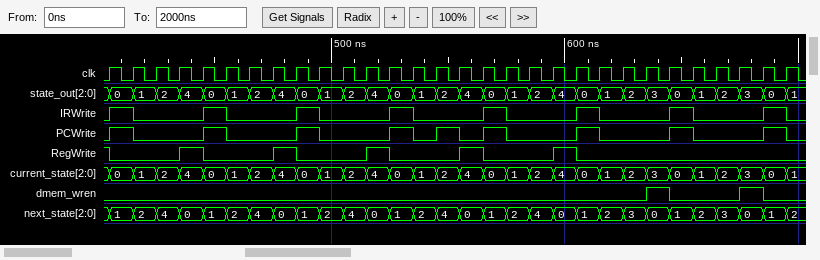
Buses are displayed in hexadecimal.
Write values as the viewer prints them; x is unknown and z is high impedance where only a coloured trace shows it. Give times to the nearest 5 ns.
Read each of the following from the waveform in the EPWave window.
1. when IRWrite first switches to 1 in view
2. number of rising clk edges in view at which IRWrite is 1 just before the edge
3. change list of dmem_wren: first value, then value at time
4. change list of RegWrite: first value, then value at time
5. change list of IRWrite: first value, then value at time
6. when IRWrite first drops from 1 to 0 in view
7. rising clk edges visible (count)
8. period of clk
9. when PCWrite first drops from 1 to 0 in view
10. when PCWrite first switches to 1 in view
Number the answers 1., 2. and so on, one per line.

1. 405 ns
2. 8
3. 0, 1 at 635 ns, 0 at 645 ns, 1 at 675 ns, 0 at 685 ns
4. 1, 0 at 405 ns, 1 at 435 ns, 0 at 445 ns, 1 at 475 ns, 0 at 485 ns, 1 at 515 ns, 0 at 525 ns, 1 at 555 ns, 0 at 565 ns, 1 at 595 ns, 0 at 605 ns
5. 0, 1 at 405 ns, 0 at 415 ns, 1 at 445 ns, 0 at 455 ns, 1 at 485 ns, 0 at 495 ns, 1 at 525 ns, 0 at 535 ns, 1 at 565 ns, 0 at 575 ns, 1 at 605 ns, 0 at 615 ns, 1 at 645 ns, 0 at 655 ns, 1 at 685 ns, 0 at 695 ns
6. 415 ns
7. 30
8. 10 ns
9. 415 ns
10. 405 ns
